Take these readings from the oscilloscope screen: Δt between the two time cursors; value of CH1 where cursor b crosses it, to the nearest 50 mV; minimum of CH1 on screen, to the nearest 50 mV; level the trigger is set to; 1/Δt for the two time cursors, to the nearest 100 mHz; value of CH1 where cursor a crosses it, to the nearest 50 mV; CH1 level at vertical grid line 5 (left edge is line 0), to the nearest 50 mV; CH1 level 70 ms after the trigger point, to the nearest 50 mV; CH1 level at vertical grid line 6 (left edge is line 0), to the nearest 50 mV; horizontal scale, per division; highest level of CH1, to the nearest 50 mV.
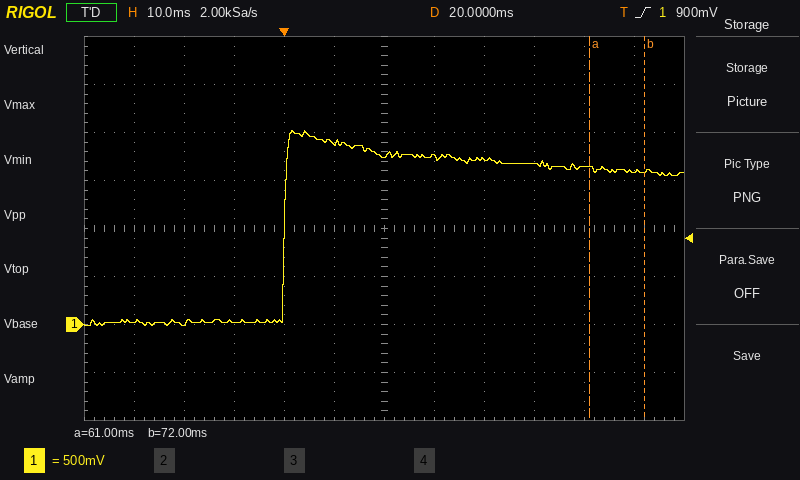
11 ms
1.60 V
0 mV
900 mV
90.9 Hz
1.65 V
1.90 V
1.60 V
1.75 V
10 ms
2.00 V
